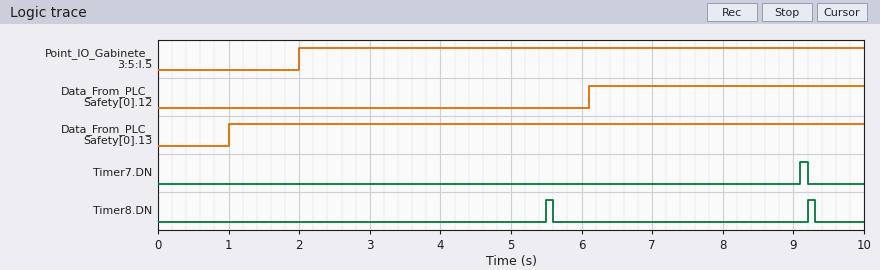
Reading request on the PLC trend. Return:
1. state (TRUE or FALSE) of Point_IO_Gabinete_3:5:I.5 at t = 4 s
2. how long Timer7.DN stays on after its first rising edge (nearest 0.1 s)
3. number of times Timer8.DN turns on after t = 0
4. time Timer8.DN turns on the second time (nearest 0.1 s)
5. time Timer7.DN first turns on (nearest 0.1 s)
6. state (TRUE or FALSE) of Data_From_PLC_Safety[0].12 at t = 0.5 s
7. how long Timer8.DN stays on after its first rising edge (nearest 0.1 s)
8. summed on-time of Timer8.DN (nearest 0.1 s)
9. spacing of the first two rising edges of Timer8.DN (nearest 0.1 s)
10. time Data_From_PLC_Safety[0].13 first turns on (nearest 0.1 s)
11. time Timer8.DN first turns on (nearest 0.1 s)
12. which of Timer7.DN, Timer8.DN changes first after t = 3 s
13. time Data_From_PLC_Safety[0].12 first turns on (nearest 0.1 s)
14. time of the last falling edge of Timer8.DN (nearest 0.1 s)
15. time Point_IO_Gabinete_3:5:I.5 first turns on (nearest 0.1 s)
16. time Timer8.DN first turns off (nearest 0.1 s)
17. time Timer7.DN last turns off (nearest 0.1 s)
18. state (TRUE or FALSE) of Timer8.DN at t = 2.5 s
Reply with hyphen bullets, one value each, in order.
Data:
- TRUE
- 0.1 s
- 2
- 9.2 s
- 9.1 s
- FALSE
- 0.1 s
- 0.2 s
- 3.7 s
- 1.0 s
- 5.5 s
- Timer8.DN
- 6.1 s
- 9.3 s
- 2.0 s
- 5.6 s
- 9.2 s
- FALSE
